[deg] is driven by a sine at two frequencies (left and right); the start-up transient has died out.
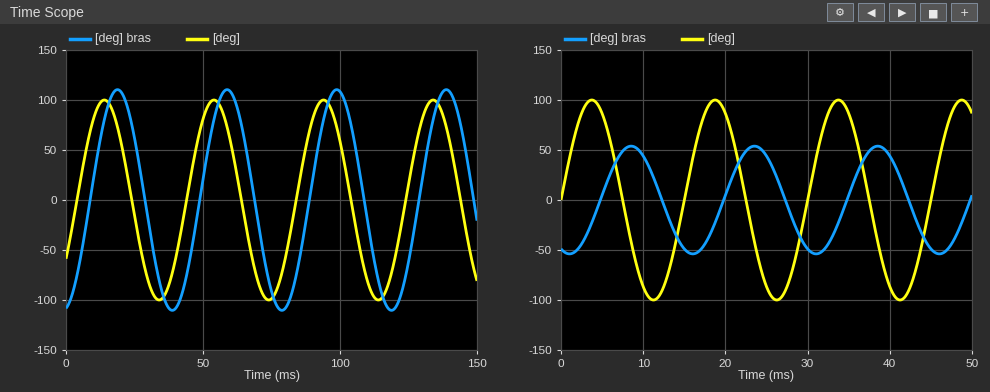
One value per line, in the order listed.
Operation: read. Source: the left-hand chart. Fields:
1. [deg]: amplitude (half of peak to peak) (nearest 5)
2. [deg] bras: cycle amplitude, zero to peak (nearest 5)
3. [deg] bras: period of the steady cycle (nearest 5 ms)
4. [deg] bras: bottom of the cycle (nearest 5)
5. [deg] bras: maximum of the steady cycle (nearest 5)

100
110
40 ms
-110
110
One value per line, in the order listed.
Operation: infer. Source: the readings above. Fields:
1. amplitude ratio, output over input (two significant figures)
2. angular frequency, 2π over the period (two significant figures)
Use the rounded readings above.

1.1
0.16 rad/ms
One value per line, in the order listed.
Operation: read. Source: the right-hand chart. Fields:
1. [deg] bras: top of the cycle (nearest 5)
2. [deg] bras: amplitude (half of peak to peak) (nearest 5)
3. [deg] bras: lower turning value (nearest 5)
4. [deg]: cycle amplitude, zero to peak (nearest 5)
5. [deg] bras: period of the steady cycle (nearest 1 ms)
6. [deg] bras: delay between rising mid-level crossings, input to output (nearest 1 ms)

55
55
-55
100
15 ms
5 ms
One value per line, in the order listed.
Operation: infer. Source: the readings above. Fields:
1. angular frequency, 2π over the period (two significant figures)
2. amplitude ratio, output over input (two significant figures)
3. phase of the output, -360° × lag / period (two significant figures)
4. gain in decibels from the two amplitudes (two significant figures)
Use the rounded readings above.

0.42 rad/ms
0.55
-120°
-5.2 dB
